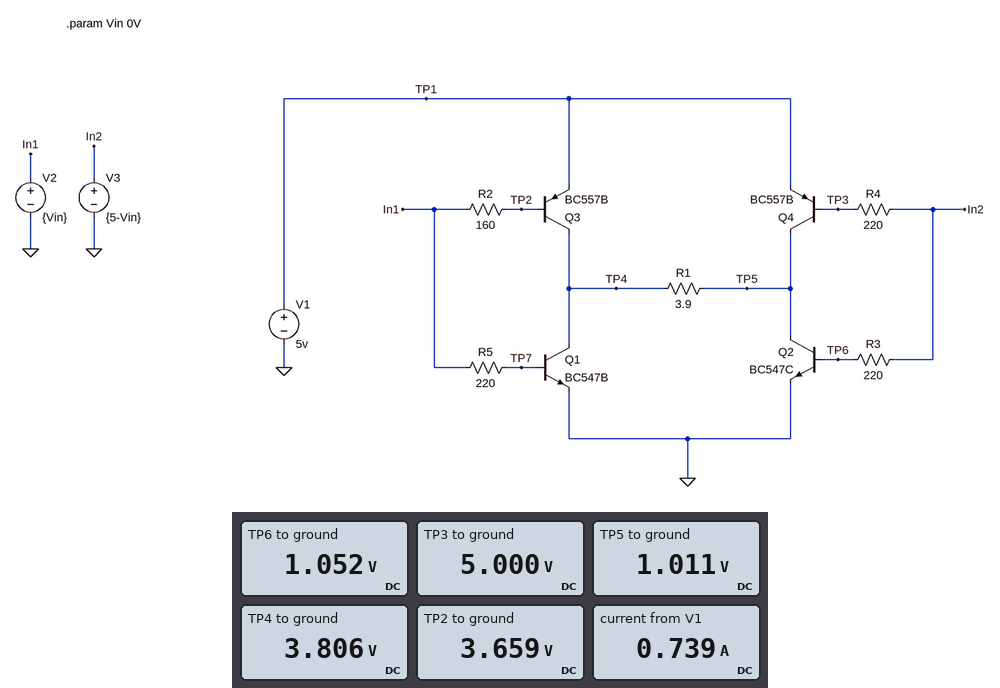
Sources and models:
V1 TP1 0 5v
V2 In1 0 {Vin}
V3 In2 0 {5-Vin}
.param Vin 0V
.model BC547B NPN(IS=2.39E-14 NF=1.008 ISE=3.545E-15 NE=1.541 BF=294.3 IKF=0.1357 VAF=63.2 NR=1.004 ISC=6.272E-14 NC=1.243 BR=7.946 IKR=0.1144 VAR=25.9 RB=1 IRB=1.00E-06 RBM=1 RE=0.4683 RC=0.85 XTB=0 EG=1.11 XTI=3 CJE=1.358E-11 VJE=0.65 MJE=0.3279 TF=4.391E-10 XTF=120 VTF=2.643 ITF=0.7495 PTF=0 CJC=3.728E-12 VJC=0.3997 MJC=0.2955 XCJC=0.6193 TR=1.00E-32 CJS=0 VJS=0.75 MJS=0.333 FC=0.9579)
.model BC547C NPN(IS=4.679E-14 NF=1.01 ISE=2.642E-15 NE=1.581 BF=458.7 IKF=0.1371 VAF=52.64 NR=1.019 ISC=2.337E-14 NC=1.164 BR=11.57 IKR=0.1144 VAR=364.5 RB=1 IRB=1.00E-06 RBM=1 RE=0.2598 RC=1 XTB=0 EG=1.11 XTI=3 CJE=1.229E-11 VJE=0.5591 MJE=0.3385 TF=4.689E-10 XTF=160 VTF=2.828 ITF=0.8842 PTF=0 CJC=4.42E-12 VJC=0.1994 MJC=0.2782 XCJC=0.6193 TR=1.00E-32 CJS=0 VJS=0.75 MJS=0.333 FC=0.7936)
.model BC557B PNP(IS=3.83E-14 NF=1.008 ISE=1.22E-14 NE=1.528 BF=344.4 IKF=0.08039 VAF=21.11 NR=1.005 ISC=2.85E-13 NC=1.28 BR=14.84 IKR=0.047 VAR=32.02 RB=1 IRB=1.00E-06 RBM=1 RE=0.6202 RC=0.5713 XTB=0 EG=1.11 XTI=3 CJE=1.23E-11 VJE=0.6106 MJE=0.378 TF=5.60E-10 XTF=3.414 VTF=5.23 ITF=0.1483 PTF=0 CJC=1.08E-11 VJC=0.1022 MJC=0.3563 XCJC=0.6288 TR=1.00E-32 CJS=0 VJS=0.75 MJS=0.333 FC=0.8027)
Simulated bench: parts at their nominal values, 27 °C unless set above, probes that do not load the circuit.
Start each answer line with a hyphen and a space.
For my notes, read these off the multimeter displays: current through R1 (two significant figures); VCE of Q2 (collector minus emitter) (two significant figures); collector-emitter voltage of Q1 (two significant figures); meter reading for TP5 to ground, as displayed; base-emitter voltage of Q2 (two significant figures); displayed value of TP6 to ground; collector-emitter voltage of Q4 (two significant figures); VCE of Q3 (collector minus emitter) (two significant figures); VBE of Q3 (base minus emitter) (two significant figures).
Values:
- 720 mA
- 1.0 V
- 3.8 V
- 1.011 V
- 1.1 V
- 1.052 V
- -4.0 V
- -1.2 V
- -1.3 V
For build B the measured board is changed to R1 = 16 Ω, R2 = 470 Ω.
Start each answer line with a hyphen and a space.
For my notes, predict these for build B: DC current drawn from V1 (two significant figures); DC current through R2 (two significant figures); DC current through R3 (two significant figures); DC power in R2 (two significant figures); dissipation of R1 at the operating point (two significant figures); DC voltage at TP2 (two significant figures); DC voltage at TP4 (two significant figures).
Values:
- 270 mA
- 8.5 mA
- 19 mA
- 34 mW
- 1.1 W
- 4.0 V
- 4.6 V
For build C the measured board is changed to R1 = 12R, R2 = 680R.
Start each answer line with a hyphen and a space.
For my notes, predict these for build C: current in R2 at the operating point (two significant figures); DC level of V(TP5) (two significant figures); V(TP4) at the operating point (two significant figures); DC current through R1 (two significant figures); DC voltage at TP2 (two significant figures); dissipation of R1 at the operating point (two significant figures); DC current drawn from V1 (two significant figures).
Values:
- 5.8 mA
- 480 mV
- 4.4 V
- 330 mA
- 4.0 V
- 1.3 W
- 340 mA
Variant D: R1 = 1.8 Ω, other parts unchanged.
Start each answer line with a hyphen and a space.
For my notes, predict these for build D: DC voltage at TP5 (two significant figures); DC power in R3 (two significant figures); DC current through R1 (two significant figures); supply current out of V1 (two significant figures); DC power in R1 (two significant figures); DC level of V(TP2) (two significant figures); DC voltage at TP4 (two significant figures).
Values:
- 1.1 V
- 70 mW
- 760 mA
- 780 mA
- 1.0 W
- 3.6 V
- 2.4 V
